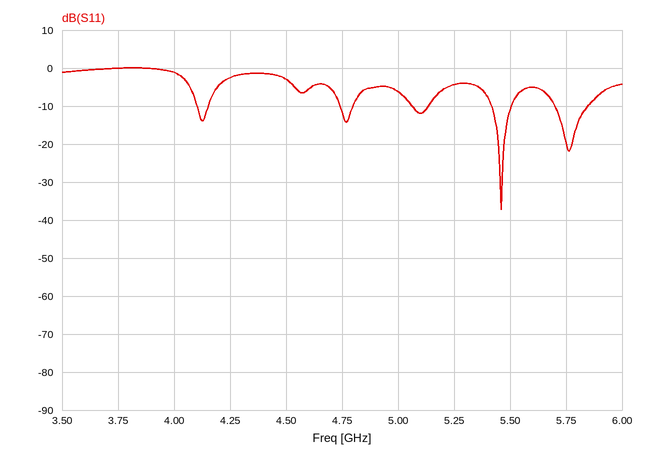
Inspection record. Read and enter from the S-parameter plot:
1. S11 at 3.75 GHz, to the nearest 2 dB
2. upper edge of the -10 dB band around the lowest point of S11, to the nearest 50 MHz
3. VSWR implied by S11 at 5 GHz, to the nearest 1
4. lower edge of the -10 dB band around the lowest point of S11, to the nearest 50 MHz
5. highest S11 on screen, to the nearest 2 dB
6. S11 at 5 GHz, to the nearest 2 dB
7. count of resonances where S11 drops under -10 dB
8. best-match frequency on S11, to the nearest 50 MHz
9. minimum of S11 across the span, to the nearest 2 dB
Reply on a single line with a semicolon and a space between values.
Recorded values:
0 dB; 5.50 GHz; 3; 5.40 GHz; 0 dB; -6 dB; 5; 5.45 GHz; -38 dB
